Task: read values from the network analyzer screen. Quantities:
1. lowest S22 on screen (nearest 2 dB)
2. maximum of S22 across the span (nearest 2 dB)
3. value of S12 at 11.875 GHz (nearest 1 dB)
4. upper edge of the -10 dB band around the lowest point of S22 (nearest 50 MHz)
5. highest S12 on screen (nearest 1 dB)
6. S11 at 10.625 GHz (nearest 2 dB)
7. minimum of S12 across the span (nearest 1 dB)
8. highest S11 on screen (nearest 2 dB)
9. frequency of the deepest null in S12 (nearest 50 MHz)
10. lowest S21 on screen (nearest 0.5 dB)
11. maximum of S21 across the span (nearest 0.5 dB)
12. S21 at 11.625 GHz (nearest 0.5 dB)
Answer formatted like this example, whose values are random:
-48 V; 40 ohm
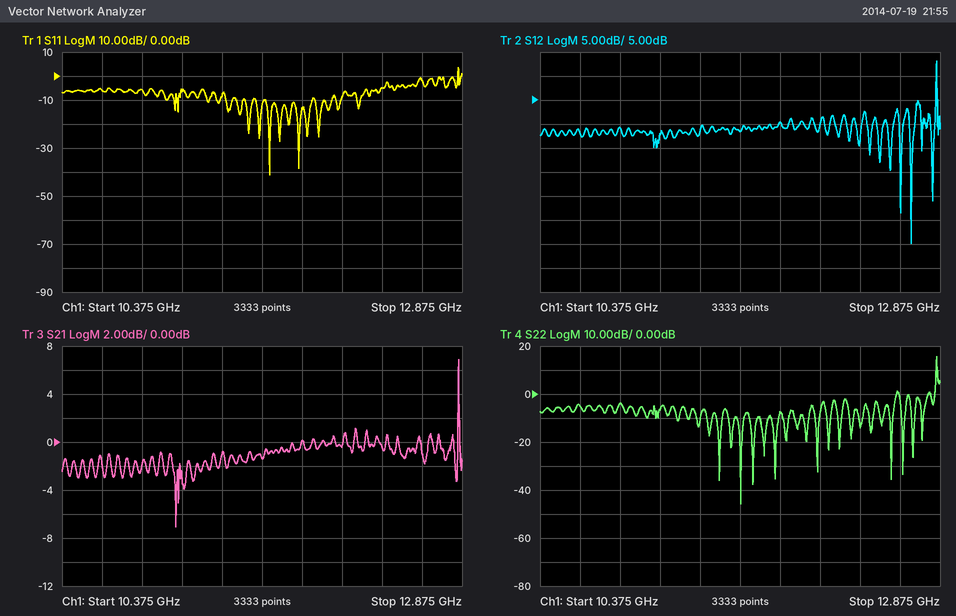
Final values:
-46 dB; 16 dB; 0 dB; 11.65 GHz; 13 dB; -6 dB; -25 dB; 4 dB; 12.70 GHz; -7.0 dB; 7.0 dB; -1.5 dB
